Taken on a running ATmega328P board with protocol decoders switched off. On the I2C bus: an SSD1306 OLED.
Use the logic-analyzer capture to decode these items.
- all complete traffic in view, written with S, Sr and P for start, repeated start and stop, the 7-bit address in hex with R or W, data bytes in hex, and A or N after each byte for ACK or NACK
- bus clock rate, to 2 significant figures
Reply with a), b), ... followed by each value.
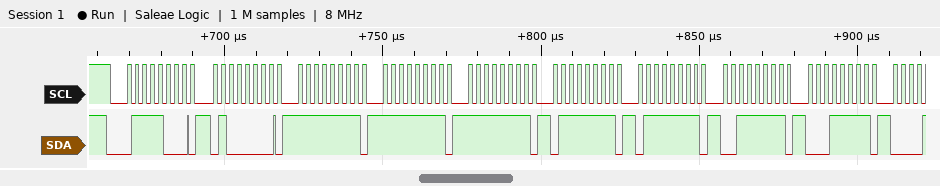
a) S 3CW A 40 A FF A FF A FF A 7F A 7F A 3F A 1F A
b) 400 kHz
